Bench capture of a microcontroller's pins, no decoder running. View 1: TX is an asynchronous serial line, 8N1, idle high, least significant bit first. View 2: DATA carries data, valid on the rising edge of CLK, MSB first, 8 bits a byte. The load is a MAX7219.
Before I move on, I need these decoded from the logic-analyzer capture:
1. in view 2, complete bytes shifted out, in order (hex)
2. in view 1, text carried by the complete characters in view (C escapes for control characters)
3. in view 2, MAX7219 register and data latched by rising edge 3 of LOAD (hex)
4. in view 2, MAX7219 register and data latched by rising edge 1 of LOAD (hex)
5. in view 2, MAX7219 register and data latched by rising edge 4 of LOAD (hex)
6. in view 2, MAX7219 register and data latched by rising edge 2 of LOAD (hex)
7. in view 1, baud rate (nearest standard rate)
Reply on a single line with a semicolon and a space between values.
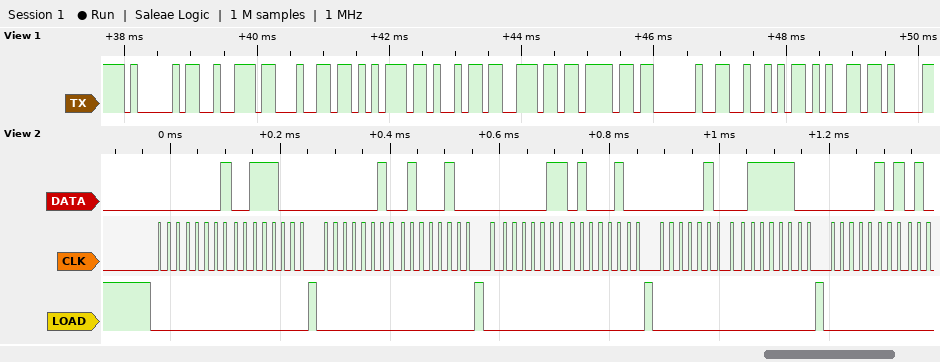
0x01 0x38 0x02 0x44 0x03 0x44 0x04 0x7C 0x05; "Arduino Re"; register 0x3, data 0x44; register 0x1, data 0x38; register 0x4, data 0x7C; register 0x2, data 0x44; 9600 baud
